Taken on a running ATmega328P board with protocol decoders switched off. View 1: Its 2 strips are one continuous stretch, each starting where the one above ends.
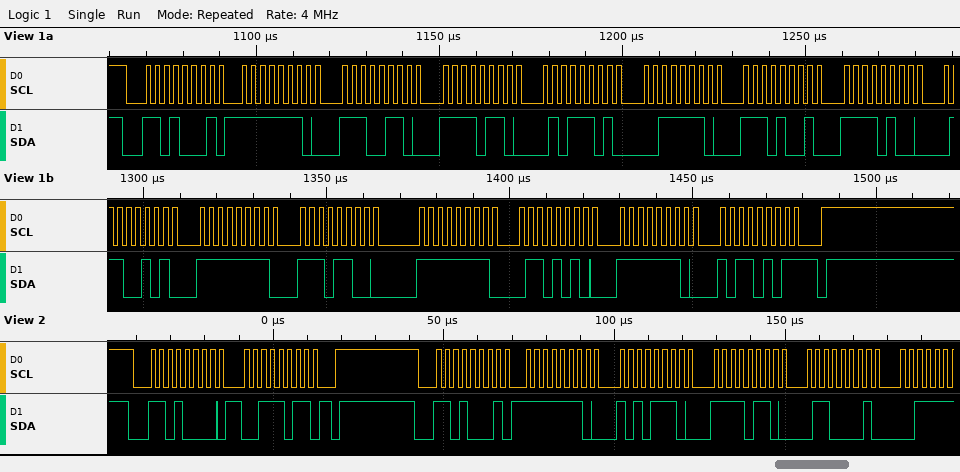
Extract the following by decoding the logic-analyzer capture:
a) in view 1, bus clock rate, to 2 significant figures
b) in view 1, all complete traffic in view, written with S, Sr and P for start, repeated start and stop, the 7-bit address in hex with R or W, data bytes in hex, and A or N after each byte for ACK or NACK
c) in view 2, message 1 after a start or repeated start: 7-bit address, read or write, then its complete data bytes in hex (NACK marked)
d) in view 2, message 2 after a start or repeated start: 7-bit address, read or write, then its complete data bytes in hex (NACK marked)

400 kHz
S 68R A FE A E6 A F6 A 5D A 3E A E9 A F4 A 65 A FF A EC A FF A 6A A FE A B5 N P
0x68 write: 3B
0x68 read: FE AE F6 61
